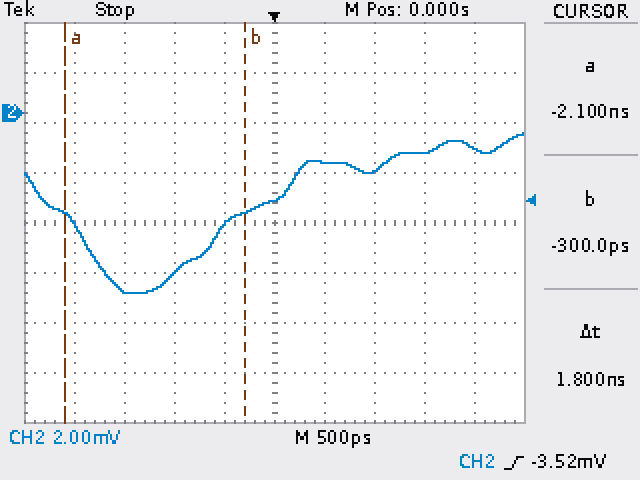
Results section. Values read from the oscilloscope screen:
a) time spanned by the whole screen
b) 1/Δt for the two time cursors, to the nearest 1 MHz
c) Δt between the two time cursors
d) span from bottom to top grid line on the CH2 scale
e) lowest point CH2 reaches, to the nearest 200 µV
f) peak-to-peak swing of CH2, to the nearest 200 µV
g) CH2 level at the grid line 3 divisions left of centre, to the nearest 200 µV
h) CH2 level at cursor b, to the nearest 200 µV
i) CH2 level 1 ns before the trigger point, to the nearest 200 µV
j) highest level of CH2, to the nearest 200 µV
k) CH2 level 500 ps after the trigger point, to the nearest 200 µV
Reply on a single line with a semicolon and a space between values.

5 ns; 556 MHz; 1.8 ns; 16 mV; -7.2 mV; 6.4 mV; -7.2 mV; -4.0 mV; -6.4 mV; -800 µV; -2.0 mV
